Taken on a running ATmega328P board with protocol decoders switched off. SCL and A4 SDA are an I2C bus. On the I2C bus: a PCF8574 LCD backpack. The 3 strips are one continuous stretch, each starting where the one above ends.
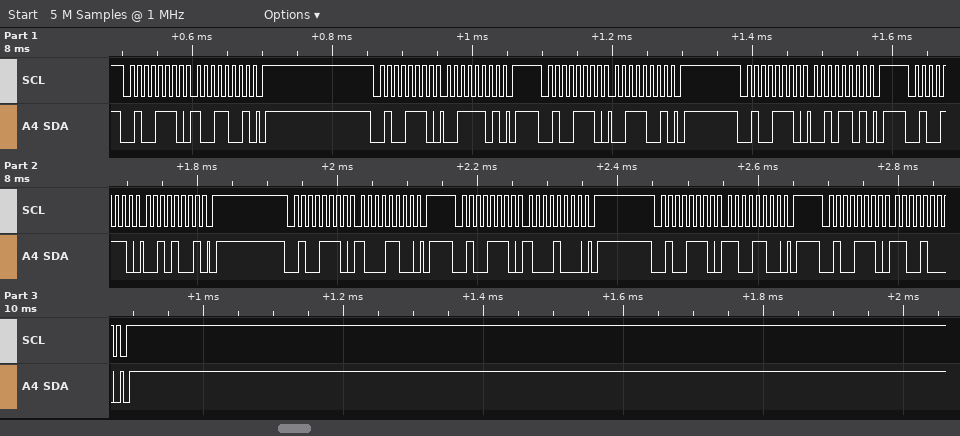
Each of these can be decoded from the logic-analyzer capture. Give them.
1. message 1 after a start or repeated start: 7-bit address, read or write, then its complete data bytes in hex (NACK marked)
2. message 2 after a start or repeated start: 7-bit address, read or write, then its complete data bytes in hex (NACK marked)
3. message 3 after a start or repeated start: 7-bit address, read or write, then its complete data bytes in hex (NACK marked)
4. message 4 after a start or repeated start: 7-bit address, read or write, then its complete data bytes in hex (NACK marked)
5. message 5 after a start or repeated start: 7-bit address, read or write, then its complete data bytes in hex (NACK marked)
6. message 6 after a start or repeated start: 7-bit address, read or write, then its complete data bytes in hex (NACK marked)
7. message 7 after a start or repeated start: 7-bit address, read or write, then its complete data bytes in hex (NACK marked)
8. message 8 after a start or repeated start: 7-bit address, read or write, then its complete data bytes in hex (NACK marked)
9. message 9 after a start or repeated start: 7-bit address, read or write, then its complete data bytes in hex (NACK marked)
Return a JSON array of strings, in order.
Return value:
["0x27 write: 99", "0x27 write: 3D", "0x27 write: 39", "0x27 write: 2D", "0x27 write: 29", "0x27 write: 8C", "0x27 write: 88", "0x27 write: CC", "0x27 write: C8"]
